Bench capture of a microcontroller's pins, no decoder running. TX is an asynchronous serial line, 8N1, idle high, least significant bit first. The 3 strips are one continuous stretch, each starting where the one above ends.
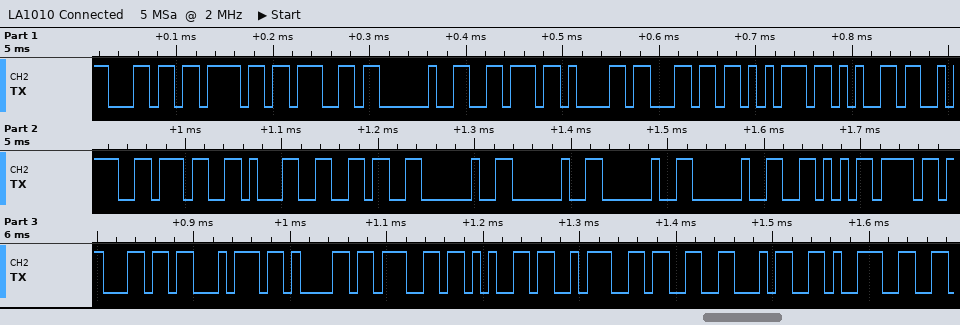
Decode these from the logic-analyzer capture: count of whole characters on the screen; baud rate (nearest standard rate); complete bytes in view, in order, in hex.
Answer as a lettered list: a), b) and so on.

a) 28
b) 115200 baud
c) 6C 6F 67 20 76 61 6C 75 65 3A 37 31 36 20 20 20 20 56 6F 6C 74 61 67 65 3A 33 34 39
